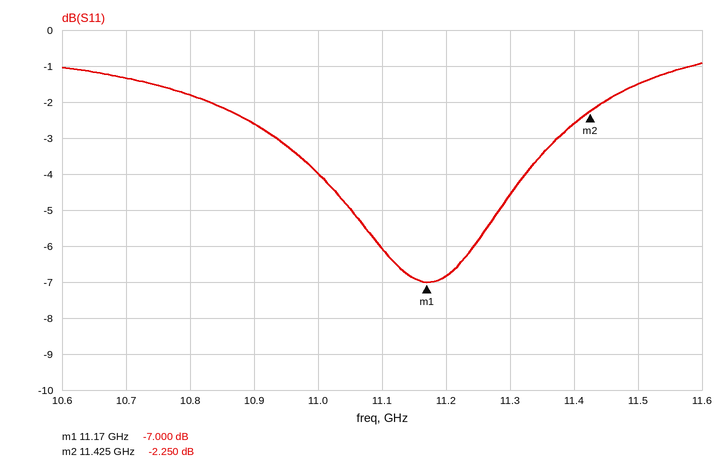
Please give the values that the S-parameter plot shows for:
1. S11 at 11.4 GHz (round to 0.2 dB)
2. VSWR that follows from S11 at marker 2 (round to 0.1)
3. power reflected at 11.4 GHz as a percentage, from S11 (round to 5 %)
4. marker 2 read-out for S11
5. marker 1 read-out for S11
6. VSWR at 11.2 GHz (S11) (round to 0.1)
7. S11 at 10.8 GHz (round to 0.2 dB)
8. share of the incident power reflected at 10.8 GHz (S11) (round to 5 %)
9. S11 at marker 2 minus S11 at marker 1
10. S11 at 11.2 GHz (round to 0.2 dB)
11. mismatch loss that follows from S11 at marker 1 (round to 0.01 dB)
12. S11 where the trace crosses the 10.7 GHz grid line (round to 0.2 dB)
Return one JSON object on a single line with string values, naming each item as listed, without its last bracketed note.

{"S11 at 11.4 GHz": "-2.6 dB", "VSWR that follows from S11 at marker 2": "7.8", "power reflected at 11.4 GHz as a percentage, from S11": "55 %", "marker 2 read-out for S11": "-2.250 dB", "marker 1 read-out for S11": "-7.000 dB", "VSWR at 11.2 GHz (S11)": "2.7", "S11 at 10.8 GHz": "-1.8 dB", "share of the incident power reflected at 10.8 GHz (S11)": "65 %", "S11 at marker 2 minus S11 at marker 1": "4.750 dB", "S11 at 11.2 GHz": "-6.8 dB", "mismatch loss that follows from S11 at marker 1": "0.97 dB", "S11 where the trace crosses the 10.7 GHz grid line": "-1.4 dB"}
